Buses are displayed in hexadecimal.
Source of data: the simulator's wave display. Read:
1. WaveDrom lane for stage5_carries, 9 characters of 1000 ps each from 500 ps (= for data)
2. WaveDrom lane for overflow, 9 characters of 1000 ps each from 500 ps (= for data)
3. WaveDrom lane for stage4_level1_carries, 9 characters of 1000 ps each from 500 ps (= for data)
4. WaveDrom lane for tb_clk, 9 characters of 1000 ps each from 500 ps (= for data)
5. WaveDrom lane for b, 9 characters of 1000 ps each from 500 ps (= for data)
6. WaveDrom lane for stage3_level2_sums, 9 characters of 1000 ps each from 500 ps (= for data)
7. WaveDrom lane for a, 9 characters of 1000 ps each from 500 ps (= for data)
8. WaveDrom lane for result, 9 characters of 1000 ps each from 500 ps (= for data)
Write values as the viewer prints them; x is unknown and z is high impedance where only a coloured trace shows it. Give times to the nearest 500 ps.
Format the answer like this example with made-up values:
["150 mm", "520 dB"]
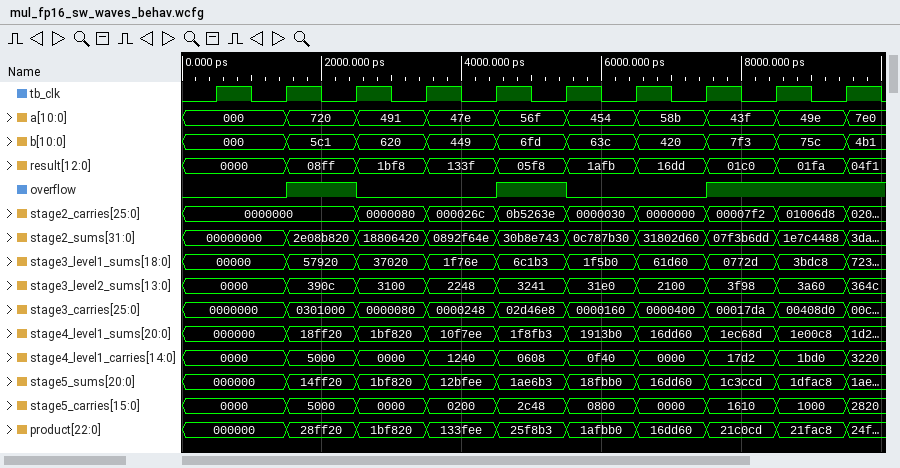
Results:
["{name: 'stage5_carries', wave: '=========', data: '0000 5000 0000 0200 2c48 0800 0000 1610 1000'}", "{name: 'overflow', wave: '010.10.1.'}", "{name: 'stage4_level1_carries', wave: '=========', data: '0000 5000 0000 1240 0608 0f40 0000 17d2 1bd0'}", "{name: 'tb_clk', wave: 'p........'}", "{name: 'b', wave: '=========', data: '000 5c1 620 449 6fd 63c 420 7f3 75c'}", "{name: 'stage3_level2_sums', wave: '=========', data: '0000 390c 3100 2248 3241 31e0 2100 3f98 3a60'}", "{name: 'a', wave: '=========', data: '000 720 491 47e 56f 454 58b 43f 49e'}", "{name: 'result', wave: '=========', data: '0000 08ff 1bf8 133f 05f8 1afb 16dd 01c0 01fa'}"]
